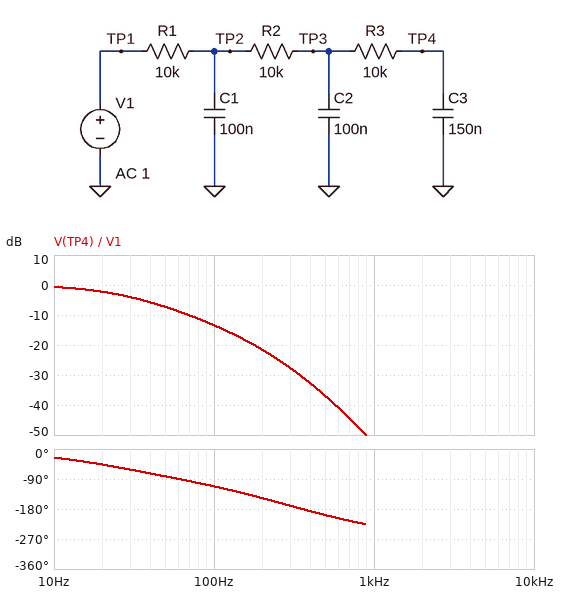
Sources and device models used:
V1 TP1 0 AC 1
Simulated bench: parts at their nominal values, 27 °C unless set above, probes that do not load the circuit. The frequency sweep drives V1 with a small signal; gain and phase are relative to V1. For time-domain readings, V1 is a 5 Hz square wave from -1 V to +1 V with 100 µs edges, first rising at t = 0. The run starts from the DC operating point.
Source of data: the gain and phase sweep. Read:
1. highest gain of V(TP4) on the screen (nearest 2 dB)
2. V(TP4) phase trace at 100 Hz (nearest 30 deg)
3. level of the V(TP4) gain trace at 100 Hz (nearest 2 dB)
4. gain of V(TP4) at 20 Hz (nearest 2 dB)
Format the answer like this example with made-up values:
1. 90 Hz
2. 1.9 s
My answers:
1. 0 dB
2. -120 deg
3. -14 dB
4. -2 dB
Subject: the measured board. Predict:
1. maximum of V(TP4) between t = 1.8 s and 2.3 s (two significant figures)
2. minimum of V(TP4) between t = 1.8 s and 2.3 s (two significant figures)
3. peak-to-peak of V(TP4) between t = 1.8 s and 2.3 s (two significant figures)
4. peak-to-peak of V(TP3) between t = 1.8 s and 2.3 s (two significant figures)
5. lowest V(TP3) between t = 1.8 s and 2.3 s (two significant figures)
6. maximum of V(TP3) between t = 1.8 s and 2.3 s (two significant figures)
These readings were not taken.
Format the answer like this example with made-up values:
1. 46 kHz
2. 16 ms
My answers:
1. 1.0 V
2. -1.0 V
3. 2.0 V
4. 2.0 V
5. -1.0 V
6. 1.0 V
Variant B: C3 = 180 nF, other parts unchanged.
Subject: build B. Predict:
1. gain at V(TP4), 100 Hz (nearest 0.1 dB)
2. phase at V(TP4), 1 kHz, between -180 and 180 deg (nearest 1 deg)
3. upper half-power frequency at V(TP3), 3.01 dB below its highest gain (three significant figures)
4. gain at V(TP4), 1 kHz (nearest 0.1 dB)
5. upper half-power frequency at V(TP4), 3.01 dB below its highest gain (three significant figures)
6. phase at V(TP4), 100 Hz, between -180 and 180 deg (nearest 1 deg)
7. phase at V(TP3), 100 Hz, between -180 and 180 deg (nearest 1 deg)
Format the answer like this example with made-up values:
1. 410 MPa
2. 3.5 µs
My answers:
1. -14.5 dB
2. 129 deg
3. 22.9 Hz
4. -54.1 dB
5. 21.5 Hz
6. -115 deg
7. -66 deg
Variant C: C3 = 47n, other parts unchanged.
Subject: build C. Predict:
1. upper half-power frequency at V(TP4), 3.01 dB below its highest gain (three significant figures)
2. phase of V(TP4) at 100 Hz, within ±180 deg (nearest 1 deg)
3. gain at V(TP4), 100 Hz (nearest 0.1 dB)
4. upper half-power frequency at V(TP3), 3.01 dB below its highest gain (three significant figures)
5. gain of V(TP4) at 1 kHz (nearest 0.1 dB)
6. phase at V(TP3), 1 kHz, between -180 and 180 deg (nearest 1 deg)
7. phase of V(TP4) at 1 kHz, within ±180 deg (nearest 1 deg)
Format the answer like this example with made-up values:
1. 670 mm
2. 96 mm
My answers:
1. 42.6 Hz
2. -93 deg
3. -8.5 dB
4. 43.2 Hz
5. -43.1 dB
6. -147 deg
7. 142 deg
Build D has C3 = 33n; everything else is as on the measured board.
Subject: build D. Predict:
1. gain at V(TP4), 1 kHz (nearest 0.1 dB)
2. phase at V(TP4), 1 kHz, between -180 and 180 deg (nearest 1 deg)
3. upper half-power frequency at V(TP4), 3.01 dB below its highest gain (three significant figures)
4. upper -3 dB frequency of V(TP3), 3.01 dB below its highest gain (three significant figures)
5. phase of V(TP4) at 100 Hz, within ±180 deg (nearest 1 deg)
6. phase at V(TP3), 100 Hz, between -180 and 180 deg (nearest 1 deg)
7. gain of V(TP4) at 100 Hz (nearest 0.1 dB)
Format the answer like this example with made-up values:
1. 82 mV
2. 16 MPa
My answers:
1. -40.6 dB
2. 148 deg
3. 46.9 Hz
4. 47.3 Hz
5. -88 deg
6. -76 deg
7. -7.7 dB
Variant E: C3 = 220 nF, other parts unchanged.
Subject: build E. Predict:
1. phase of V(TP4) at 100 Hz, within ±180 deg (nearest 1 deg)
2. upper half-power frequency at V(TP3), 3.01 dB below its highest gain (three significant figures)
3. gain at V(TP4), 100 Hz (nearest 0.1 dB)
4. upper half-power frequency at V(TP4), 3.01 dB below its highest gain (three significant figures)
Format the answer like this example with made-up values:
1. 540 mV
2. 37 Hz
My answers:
1. -118 deg
2. 19.9 Hz
3. -15.8 dB
4. 18.6 Hz
